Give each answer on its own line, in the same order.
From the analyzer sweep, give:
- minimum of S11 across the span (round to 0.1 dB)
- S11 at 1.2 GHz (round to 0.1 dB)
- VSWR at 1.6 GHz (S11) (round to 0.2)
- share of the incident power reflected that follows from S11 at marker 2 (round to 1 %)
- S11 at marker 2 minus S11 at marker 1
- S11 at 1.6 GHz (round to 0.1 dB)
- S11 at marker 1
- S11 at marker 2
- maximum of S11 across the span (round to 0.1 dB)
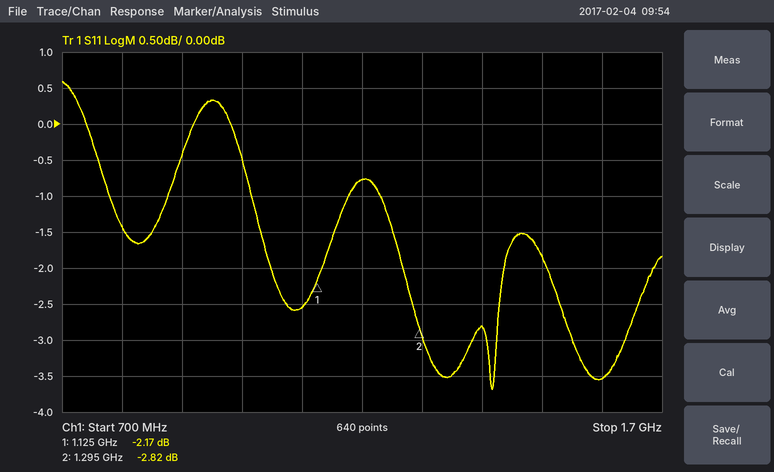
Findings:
-3.7 dB
-0.8 dB
5.0
52 %
-0.65 dB
-3.5 dB
-2.17 dB
-2.82 dB
0.6 dB
